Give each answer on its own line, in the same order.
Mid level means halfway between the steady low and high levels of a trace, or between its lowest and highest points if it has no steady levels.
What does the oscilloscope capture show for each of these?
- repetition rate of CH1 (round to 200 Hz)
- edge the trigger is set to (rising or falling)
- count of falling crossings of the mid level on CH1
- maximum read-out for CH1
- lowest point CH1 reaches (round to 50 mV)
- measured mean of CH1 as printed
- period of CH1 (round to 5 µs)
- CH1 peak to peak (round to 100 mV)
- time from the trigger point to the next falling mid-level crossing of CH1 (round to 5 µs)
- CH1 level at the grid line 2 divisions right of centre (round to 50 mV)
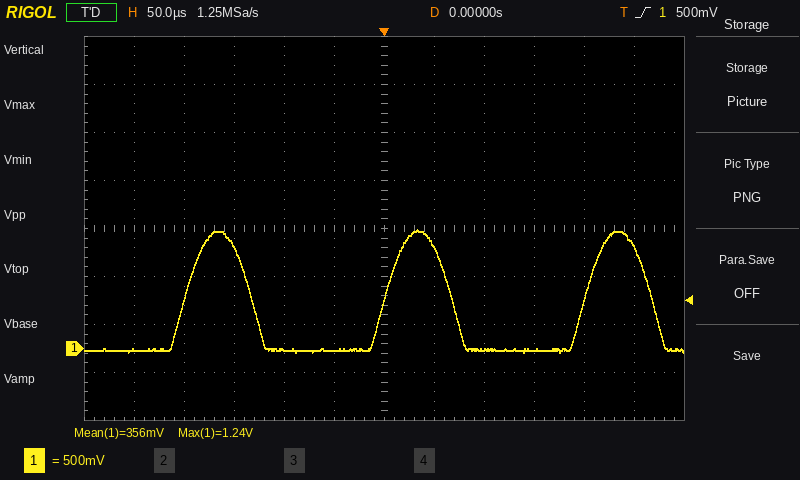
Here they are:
5.0 kHz
rising
3
1.24 V
-50 mV
356 mV
200 µs
1.30 V
65 µs
0 mV
